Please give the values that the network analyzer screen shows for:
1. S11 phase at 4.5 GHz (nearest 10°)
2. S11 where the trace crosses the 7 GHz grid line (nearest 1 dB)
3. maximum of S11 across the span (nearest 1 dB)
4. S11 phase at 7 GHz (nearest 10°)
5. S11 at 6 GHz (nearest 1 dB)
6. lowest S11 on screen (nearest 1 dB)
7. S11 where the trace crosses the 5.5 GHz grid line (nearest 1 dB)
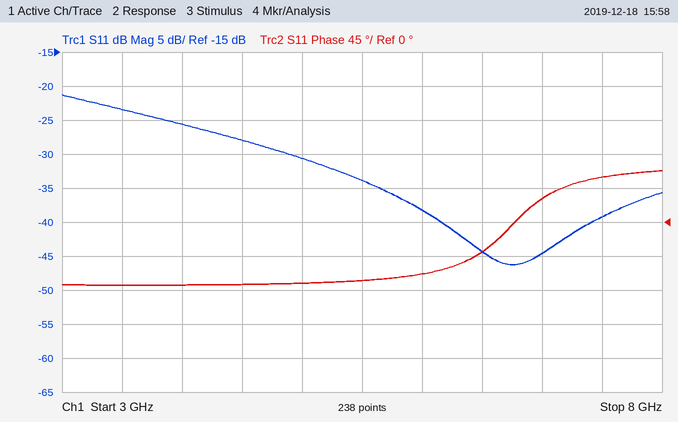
-80°
-45 dB
-21 dB
30°
-38 dB
-46 dB
-34 dB
